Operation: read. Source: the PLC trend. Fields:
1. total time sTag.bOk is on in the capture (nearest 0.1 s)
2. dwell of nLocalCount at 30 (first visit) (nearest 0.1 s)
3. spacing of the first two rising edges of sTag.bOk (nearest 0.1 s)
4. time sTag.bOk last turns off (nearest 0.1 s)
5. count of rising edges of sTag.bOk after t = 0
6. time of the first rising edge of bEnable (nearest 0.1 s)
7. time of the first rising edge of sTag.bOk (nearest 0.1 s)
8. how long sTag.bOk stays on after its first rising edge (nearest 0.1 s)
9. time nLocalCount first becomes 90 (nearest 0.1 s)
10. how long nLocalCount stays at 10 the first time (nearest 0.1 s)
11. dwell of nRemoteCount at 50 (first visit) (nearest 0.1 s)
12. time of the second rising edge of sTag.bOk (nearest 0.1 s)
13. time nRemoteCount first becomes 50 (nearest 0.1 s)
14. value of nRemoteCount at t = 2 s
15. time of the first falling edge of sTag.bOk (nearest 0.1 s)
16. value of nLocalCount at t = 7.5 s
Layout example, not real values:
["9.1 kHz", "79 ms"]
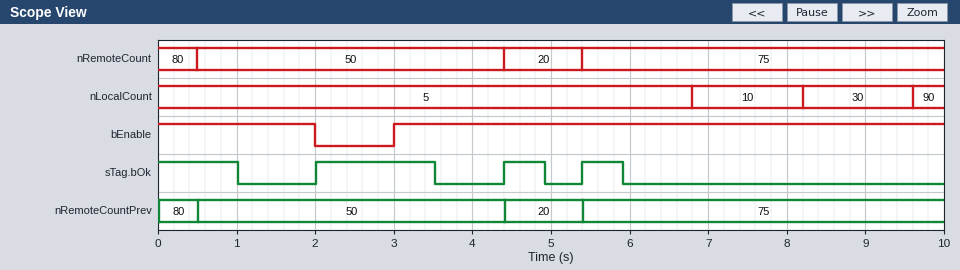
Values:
["3.6 s", "1.4 s", "2.4 s", "5.9 s", "3", "3.0 s", "2.0 s", "1.5 s", "9.6 s", "1.4 s", "3.9 s", "4.4 s", "0.5 s", "50", "1.0 s", "10"]
